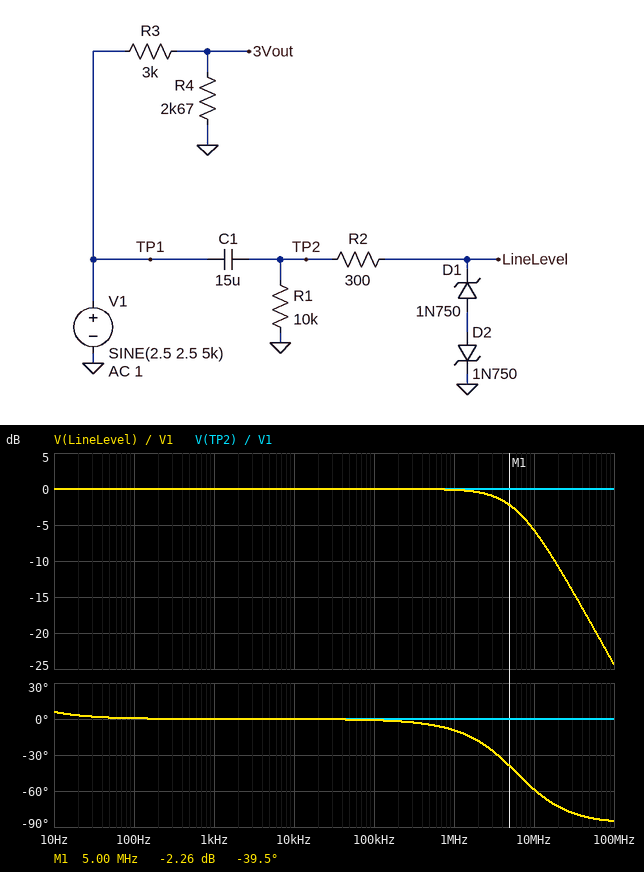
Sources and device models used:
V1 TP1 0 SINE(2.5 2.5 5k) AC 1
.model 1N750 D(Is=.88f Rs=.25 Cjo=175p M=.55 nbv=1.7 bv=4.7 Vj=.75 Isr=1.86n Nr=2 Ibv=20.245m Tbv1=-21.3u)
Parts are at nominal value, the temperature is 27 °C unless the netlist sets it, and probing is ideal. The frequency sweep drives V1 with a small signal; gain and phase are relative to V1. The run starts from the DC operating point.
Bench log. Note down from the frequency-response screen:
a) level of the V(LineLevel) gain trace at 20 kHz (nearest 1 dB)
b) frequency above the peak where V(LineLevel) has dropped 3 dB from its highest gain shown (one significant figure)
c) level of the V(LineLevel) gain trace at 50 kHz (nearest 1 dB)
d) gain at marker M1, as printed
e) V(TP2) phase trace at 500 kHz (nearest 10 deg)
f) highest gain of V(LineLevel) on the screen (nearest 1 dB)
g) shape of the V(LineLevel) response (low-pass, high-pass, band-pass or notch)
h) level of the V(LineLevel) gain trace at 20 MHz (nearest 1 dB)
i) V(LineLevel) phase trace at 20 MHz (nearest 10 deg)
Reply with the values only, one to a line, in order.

0 dB
6 MHz
0 dB
-2.26 dB
0 deg
0 dB
low-pass
-11 dB
-70 deg
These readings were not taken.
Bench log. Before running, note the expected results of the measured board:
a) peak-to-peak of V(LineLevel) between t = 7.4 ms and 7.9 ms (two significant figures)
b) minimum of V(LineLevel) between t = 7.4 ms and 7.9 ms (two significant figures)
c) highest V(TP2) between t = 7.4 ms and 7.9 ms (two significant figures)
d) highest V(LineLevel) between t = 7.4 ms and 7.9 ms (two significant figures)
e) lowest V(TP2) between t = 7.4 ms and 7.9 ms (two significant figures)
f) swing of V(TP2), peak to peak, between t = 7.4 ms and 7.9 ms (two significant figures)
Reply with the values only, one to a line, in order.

5.0 V
-2.5 V
2.5 V
2.5 V
-2.5 V
5.0 V
